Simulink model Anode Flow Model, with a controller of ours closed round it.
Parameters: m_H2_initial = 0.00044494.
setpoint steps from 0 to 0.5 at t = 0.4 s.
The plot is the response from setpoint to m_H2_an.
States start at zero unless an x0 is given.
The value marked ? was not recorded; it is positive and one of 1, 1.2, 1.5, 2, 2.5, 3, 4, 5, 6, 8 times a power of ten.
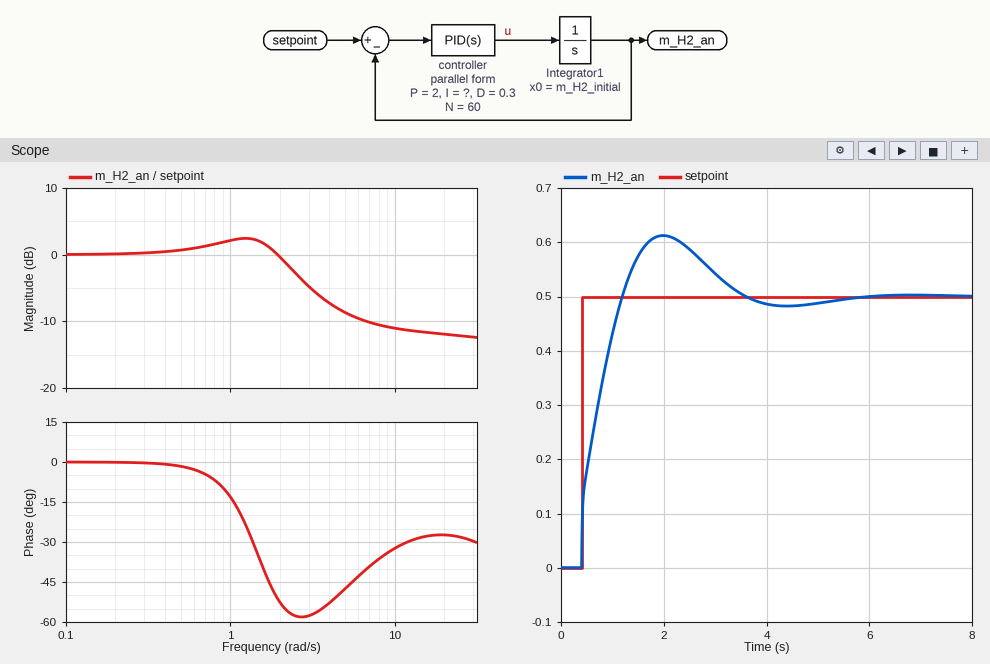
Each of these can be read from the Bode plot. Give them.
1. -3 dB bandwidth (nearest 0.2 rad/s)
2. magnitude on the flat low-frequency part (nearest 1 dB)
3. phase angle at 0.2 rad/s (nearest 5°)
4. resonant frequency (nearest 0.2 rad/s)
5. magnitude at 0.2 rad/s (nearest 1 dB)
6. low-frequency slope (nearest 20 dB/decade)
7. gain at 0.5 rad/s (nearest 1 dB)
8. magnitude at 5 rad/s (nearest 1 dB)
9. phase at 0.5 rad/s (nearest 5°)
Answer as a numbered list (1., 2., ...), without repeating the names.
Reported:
1. 2.6 rad/s
2. 0 dB
3. 0°
4. 1.2 rad/s
5. 0 dB
6. 0 dB/decade
7. 1 dB
8. -9 dB
9. 0°
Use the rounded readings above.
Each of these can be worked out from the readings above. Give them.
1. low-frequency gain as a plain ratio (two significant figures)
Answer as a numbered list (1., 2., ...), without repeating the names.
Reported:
1. 1.0
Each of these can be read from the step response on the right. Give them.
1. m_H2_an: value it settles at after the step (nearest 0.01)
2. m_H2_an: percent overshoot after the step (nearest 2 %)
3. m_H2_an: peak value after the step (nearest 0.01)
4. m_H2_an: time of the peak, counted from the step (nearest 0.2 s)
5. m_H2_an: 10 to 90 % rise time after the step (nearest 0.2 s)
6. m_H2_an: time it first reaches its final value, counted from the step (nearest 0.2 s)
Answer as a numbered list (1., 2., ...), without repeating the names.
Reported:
1. 0.50
2. 22 %
3. 0.61
4. 1.6 s
5. 0.6 s
6. 0.8 s
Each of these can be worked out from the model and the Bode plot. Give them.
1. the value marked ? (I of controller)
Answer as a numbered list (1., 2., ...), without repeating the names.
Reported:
1. 3
